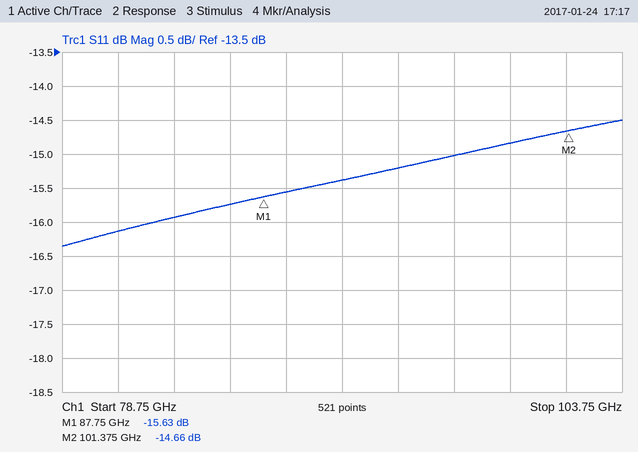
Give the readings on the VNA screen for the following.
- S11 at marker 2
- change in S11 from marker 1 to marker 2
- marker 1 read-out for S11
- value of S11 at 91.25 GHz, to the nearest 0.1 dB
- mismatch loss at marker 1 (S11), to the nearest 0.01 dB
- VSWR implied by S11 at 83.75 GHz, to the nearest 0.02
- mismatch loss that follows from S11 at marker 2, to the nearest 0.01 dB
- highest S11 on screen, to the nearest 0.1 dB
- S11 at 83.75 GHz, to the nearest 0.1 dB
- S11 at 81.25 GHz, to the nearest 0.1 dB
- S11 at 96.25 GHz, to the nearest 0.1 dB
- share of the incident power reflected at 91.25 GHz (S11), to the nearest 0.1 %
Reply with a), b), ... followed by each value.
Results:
a) -14.66 dB
b) 0.97 dB
c) -15.63 dB
d) -15.4 dB
e) 0.12 dB
f) 1.38
g) 0.15 dB
h) -14.5 dB
i) -15.9 dB
j) -16.1 dB
k) -15.0 dB
l) 2.9 %
